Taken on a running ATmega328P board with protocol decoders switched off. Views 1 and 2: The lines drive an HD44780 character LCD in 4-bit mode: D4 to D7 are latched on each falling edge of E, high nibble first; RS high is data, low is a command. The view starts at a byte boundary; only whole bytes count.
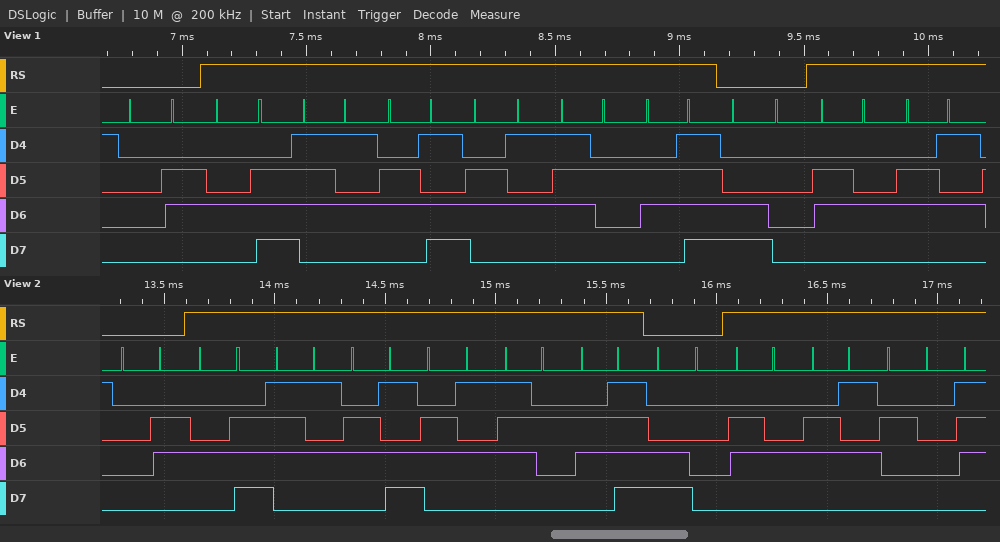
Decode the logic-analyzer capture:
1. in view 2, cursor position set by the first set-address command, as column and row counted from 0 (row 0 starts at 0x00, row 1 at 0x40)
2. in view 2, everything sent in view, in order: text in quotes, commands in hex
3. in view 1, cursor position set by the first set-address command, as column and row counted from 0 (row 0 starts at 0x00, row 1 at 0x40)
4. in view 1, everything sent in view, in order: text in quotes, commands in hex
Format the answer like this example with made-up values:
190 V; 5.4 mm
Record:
column 0, row 1; 0x06 "Numero" 0xC0 "de "; column 0, row 1; 0x06 "Numero" 0xC0 "de"
